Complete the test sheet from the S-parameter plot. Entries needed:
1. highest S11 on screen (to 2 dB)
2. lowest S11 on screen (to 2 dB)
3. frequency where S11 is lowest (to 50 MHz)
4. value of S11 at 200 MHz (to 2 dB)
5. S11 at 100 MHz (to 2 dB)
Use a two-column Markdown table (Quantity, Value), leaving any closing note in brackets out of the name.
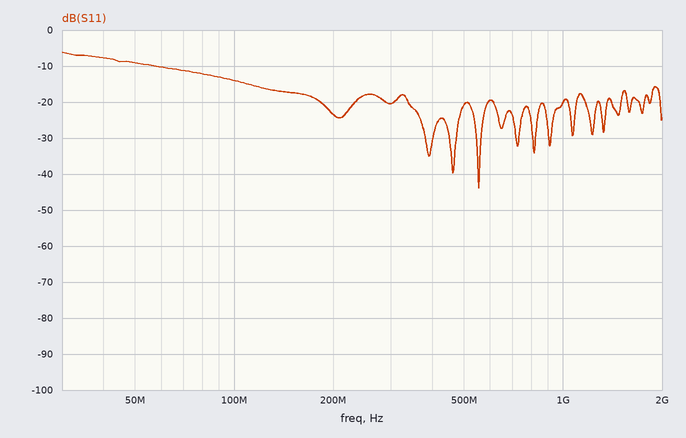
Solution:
| Quantity | Value |
|---|---|
| highest S11 on screen | -6 dB |
| lowest S11 on screen | -44 dB |
| frequency where S11 is lowest | 550 MHz |
| value of S11 at 200 MHz | -24 dB |
| S11 at 100 MHz | -14 dB |
